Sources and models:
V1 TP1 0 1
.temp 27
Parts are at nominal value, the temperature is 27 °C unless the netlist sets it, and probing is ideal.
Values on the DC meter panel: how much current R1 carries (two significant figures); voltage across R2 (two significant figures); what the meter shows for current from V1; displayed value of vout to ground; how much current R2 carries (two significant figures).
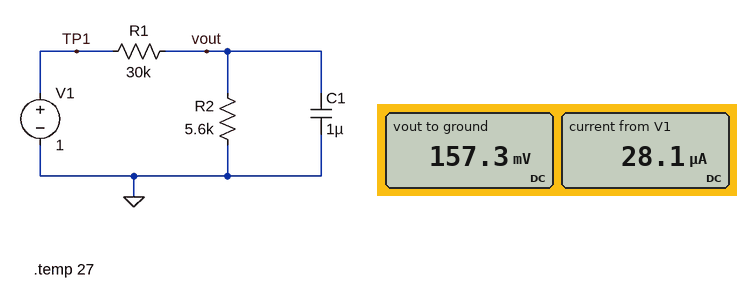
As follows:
28 µA
160 mV
28.1 µA
157.3 mV
28 µA
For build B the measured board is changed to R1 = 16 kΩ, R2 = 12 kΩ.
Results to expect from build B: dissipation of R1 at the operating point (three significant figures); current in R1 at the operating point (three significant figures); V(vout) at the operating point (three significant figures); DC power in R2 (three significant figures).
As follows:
20.4 µW
35.7 µA
429 mV
15.3 µW
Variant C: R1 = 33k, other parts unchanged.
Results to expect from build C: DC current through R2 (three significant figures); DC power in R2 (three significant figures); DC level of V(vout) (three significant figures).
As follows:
25.9 µA
3.76 µW
145 mV
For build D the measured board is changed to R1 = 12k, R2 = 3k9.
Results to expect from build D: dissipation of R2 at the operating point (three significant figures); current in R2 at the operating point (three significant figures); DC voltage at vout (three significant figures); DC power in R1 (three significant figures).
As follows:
15.4 µW
62.9 µA
245 mV
47.5 µW
